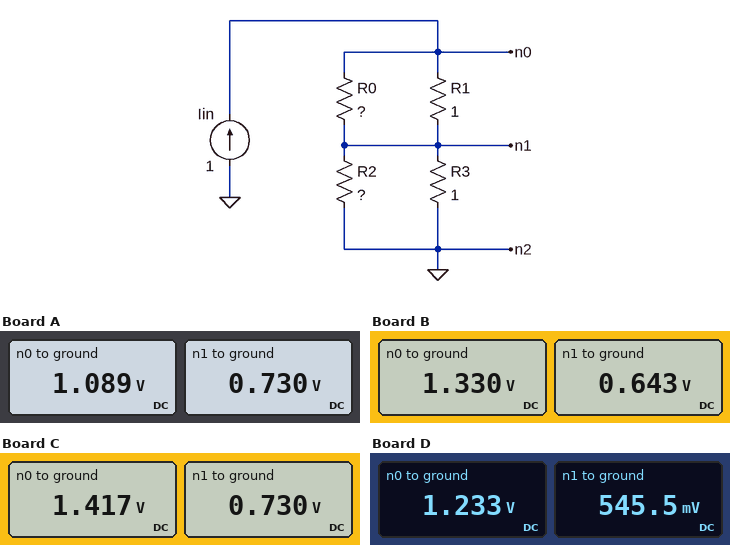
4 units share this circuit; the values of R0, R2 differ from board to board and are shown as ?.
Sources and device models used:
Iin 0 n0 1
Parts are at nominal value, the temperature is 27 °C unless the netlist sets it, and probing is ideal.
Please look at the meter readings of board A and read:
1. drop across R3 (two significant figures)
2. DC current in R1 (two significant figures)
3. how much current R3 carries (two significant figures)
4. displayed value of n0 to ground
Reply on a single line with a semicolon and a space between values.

730 mV; 360 mA; 730 mA; 1.089 V
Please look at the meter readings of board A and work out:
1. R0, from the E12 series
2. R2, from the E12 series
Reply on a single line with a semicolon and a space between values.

0.56 Ω; 2.7 Ω
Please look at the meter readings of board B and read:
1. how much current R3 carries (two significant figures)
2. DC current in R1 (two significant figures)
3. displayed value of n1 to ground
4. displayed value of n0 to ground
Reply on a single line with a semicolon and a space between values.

640 mA; 690 mA; 0.643 V; 1.330 V
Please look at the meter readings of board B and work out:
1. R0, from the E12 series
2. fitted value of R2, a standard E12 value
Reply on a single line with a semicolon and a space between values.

2.2 Ω; 1.8 Ω
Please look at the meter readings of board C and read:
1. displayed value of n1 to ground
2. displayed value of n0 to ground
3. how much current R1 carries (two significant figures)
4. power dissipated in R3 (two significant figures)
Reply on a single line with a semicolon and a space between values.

0.730 V; 1.417 V; 690 mA; 530 mW
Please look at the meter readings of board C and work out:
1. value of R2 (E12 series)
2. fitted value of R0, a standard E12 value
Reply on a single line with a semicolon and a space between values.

2.7 Ω; 2.2 Ω
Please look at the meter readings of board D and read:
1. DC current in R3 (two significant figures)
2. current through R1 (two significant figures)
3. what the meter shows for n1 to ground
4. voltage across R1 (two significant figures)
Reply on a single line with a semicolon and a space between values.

550 mA; 690 mA; 545.5 mV; 690 mV
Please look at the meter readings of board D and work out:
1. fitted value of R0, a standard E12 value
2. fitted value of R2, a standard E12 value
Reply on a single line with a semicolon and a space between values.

2.2 Ω; 1.2 Ω
